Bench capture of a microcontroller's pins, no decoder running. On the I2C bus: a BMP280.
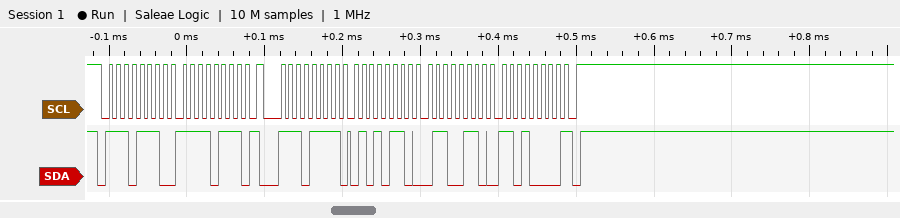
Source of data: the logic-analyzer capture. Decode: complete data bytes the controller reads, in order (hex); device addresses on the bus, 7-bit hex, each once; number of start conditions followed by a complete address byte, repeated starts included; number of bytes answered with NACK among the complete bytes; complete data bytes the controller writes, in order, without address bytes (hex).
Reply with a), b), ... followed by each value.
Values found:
a) 56 66 D0
b) 0x77
c) 2
d) 1
e) F7
